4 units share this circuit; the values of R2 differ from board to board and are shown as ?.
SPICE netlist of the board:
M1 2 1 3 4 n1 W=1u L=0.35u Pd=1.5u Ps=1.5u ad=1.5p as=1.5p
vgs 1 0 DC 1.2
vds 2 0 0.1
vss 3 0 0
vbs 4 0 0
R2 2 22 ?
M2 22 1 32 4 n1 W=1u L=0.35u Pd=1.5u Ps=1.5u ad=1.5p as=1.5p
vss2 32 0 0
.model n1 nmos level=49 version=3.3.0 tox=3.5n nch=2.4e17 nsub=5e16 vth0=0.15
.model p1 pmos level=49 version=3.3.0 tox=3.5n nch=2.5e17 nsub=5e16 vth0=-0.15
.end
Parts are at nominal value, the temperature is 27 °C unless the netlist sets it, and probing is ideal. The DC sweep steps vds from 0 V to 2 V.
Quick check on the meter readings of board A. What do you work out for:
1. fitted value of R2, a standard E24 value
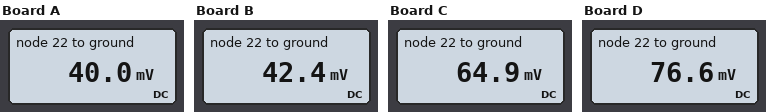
2.2 kΩ
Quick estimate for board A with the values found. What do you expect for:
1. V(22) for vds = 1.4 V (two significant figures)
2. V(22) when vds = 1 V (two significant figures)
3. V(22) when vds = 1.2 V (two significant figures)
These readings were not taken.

970 mV
590 mV
780 mV
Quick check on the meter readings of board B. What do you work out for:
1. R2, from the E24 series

2 kΩ
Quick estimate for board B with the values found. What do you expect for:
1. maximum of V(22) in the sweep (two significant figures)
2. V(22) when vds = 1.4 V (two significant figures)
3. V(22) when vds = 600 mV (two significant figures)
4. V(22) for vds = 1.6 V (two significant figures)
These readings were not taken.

1.6 V
1.0 V
310 mV
1.2 V
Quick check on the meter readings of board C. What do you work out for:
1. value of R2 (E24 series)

820 Ω
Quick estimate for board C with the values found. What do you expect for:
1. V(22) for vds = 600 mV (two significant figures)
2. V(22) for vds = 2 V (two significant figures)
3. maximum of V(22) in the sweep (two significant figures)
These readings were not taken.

460 mV
1.8 V
1.8 V
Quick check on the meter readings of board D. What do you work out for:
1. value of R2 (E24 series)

470 Ω
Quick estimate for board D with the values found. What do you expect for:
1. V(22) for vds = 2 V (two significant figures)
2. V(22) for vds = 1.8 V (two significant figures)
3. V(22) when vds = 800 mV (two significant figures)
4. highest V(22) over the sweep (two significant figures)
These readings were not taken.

1.9 V
1.7 V
710 mV
1.9 V
